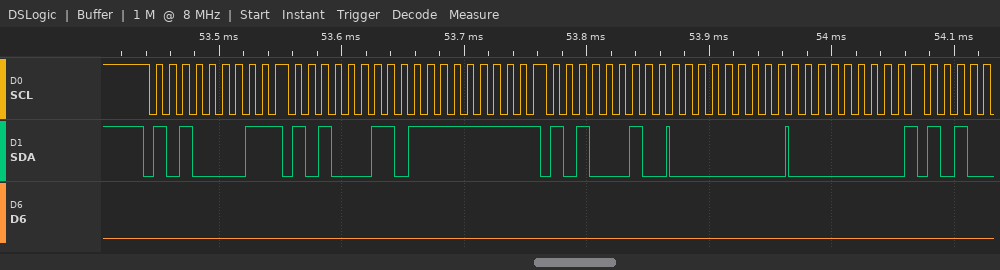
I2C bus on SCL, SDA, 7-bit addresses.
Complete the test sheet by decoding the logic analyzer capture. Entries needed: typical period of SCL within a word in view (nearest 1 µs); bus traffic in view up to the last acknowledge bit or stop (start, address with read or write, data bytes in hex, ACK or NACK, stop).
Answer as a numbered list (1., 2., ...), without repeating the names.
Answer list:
1. 11 µs
2. start, address 50 read NACK, repeated start, address 51 read ACK, FF NACK, repeated start, address 51 write ACK, 00 ACK, 00 ACK
